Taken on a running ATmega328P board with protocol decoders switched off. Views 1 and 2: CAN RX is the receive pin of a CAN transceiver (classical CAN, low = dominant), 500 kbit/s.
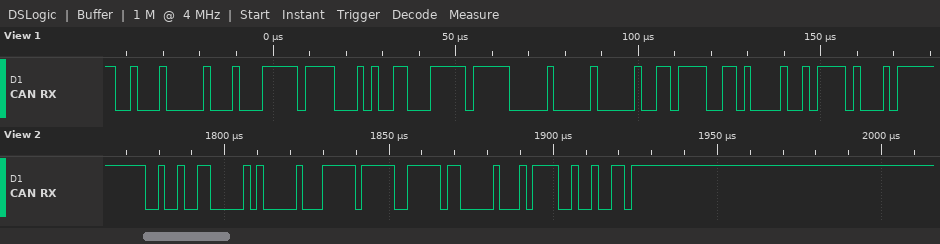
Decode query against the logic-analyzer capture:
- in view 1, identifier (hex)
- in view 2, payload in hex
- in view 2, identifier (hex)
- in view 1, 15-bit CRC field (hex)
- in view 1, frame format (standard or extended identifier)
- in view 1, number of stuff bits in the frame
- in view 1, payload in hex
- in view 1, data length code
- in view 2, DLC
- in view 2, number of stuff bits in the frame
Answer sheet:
0x220
03 FF 7F 00
0x24C
0x25E8
standard
7
FF 8A 63 FF 00 00 DE 68
8
4
6
